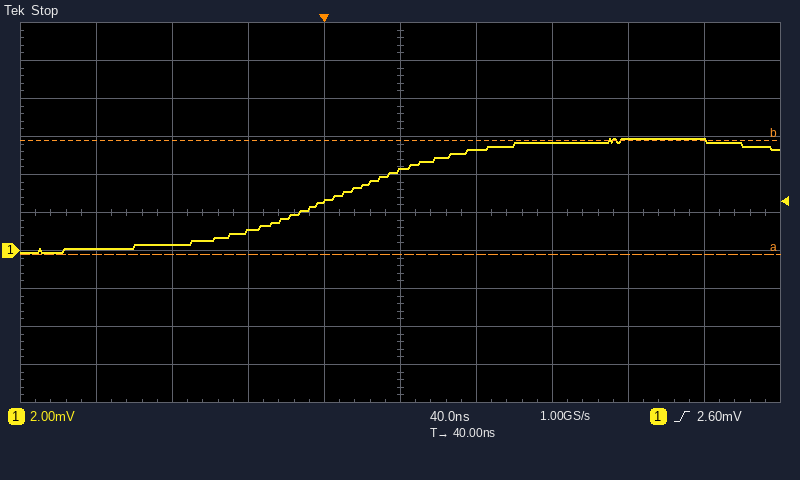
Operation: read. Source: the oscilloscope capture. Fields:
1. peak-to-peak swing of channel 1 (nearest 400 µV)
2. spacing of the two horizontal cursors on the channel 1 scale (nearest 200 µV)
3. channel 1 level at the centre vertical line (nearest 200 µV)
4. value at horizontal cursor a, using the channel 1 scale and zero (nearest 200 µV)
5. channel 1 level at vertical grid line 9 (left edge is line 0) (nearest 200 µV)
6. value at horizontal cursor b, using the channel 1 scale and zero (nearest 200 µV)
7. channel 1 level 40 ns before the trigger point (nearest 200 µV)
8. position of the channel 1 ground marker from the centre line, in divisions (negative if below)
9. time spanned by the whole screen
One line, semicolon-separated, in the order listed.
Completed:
6.0 mV; 6.0 mV; 4.2 mV; -200 µV; 5.8 mV; 5.8 mV; 1.0 mV; -1.0 div; 400 ns
